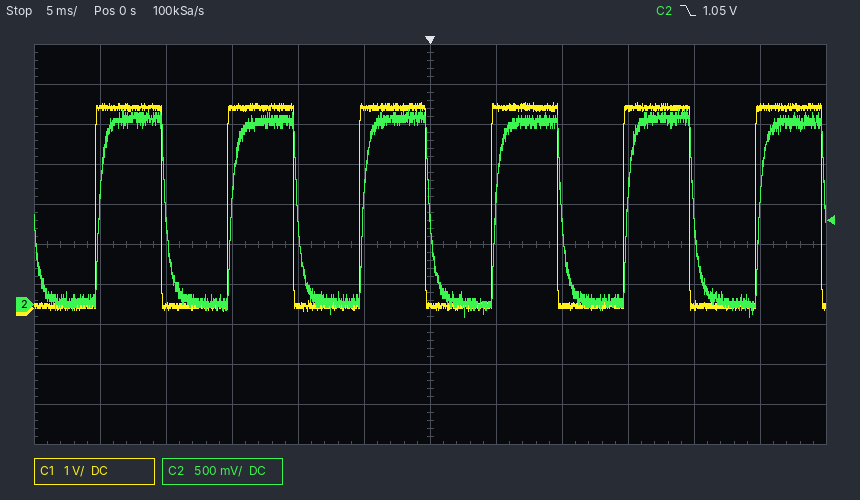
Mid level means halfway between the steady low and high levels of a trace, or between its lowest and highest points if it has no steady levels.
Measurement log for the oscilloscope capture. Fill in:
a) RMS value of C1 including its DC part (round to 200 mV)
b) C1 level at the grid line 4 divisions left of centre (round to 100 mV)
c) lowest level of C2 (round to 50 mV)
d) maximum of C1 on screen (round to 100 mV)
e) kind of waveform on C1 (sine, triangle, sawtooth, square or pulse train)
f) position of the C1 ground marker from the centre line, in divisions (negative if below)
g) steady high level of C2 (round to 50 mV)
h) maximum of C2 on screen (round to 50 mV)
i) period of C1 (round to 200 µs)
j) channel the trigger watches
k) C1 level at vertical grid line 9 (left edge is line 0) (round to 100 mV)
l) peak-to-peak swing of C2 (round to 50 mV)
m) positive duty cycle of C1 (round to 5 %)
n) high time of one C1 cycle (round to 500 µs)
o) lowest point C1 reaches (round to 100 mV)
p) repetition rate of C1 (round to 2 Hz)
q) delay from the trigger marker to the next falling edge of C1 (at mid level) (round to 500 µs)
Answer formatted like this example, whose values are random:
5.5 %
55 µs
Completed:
3.6 V
100 mV
-150 mV
5.2 V
square
-1.6 div
2.30 V
2.45 V
10.0 ms
C2
5.0 V
2.60 V
50 %
5.0 ms
-100 mV
100 Hz
9.5 ms
